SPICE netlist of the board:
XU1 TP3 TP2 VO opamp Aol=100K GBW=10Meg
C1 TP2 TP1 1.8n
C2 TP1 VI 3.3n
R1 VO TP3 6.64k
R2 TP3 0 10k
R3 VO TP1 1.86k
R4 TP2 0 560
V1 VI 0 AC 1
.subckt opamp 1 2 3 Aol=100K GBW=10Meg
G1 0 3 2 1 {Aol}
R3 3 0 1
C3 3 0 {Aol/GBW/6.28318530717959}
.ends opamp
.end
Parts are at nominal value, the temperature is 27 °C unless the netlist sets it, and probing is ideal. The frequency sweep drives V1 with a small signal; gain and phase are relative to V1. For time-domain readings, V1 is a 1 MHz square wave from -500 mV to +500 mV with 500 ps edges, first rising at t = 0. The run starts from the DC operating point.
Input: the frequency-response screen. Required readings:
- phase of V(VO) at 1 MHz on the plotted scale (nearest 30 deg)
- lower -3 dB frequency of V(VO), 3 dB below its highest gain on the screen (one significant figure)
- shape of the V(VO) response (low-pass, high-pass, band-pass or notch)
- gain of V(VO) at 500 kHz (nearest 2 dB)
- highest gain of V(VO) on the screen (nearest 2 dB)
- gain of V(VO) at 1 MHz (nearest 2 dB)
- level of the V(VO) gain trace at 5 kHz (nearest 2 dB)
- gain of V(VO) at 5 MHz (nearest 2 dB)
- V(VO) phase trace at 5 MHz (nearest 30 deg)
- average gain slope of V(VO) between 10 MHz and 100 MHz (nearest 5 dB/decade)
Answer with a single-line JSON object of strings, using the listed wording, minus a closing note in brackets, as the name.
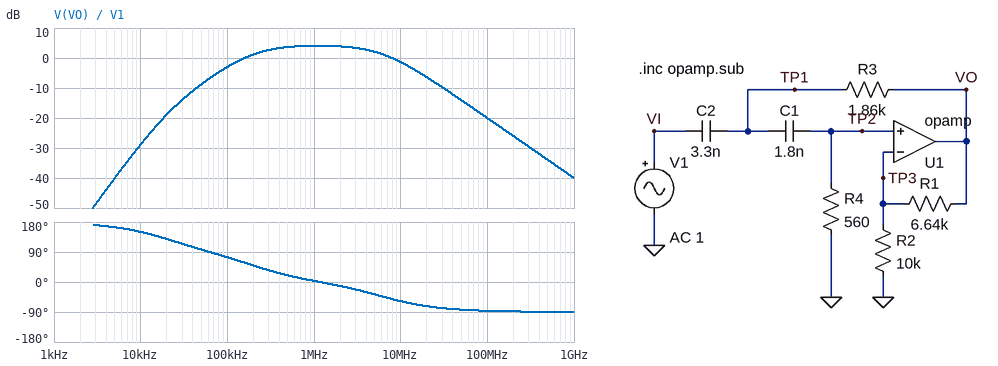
{"phase of V(VO) at 1 MHz on the plotted scale": "0 deg", "lower -3 dB frequency of V(VO), 3 dB below its highest gain on the screen": "200 kHz", "shape of the V(VO) response": "band-pass", "gain of V(VO) at 500 kHz": "4 dB", "highest gain of V(VO) on the screen": "4 dB", "gain of V(VO) at 1 MHz": "4 dB", "level of the V(VO) gain trace at 5 kHz": "-40 dB", "gain of V(VO) at 5 MHz": "2 dB", "V(VO) phase trace at 5 MHz": "-30 deg", "average gain slope of V(VO) between 10 MHz and 100 MHz": "-20 dB/decade"}
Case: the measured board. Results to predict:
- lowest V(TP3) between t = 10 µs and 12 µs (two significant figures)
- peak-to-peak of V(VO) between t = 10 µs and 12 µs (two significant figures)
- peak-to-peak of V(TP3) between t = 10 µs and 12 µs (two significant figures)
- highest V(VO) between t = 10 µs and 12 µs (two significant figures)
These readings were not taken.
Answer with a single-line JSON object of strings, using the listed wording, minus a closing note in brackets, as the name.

{"lowest V(TP3) between t = 10 µs and 12 µs": "-590 mV", "peak-to-peak of V(VO) between t = 10 µs and 12 µs": "1.9 V", "peak-to-peak of V(TP3) between t = 10 µs and 12 µs": "1.2 V", "highest V(VO) between t = 10 µs and 12 µs": "940 mV"}
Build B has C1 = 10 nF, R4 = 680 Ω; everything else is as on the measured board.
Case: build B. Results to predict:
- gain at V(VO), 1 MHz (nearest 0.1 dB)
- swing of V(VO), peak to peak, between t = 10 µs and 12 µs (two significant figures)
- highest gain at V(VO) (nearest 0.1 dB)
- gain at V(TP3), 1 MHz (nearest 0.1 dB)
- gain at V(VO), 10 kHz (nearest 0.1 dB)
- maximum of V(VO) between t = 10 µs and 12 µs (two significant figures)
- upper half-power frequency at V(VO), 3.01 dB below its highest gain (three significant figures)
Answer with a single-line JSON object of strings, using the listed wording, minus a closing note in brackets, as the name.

{"gain at V(VO), 1 MHz": "4.2 dB", "swing of V(VO), peak to peak, between t = 10 µs and 12 µs": "1.7 V", "highest gain at V(VO)": "4.3 dB", "gain at V(TP3), 1 MHz": "-0.2 dB", "gain at V(VO), 10 kHz": "-14.9 dB", "maximum of V(VO) between t = 10 µs and 12 µs": "810 mV", "upper half-power frequency at V(VO), 3.01 dB below its highest gain": "6.19 MHz"}
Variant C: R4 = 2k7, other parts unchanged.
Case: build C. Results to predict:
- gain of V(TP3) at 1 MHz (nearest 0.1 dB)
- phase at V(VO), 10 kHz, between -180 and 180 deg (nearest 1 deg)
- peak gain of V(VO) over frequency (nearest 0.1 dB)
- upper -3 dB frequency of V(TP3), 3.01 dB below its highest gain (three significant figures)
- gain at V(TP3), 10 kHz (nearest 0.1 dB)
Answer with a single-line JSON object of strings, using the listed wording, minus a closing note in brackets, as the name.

{"gain of V(TP3) at 1 MHz": "-0.2 dB", "phase at V(VO), 10 kHz, between -180 and 180 deg": "156 deg", "peak gain of V(VO) over frequency": "4.9 dB", "upper -3 dB frequency of V(TP3), 3.01 dB below its highest gain": "5.27 MHz", "gain at V(TP3), 10 kHz": "-18.3 dB"}
